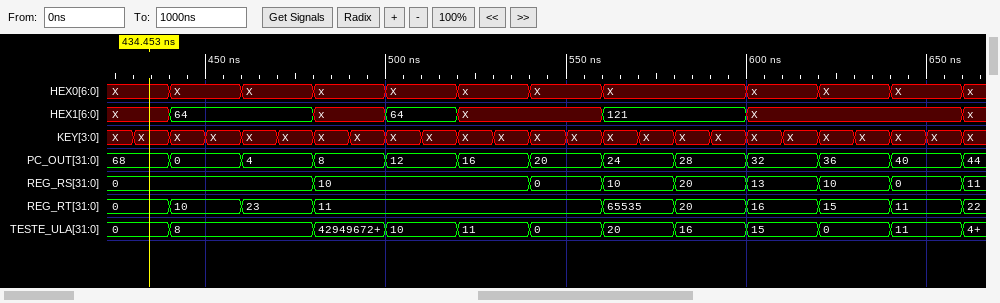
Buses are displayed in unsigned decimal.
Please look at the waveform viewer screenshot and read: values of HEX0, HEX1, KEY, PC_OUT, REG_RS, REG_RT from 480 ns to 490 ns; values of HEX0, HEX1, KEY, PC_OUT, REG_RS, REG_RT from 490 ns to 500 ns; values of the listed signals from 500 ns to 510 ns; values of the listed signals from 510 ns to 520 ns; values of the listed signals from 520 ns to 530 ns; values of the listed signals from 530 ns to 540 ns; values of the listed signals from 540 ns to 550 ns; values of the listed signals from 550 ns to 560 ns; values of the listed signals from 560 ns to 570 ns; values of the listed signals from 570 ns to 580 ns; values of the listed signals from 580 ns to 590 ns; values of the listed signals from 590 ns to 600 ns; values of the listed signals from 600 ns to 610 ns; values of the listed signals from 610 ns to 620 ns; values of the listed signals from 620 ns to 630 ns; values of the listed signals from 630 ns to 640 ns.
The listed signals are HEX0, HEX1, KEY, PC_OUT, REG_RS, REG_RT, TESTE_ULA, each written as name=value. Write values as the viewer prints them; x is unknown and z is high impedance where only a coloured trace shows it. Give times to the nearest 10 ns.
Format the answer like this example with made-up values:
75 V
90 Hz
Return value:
HEX0=x, HEX1=x, KEY=X, PC_OUT=8, REG_RS=10, REG_RT=11
HEX0=x, HEX1=x, KEY=X, PC_OUT=8, REG_RS=10, REG_RT=11
HEX0=X, HEX1=64, KEY=X, PC_OUT=12, REG_RS=10, REG_RT=11, TESTE_ULA=10
HEX0=X, HEX1=64, KEY=X, PC_OUT=12, REG_RS=10, REG_RT=11, TESTE_ULA=10
HEX0=x, HEX1=X, KEY=X, PC_OUT=16, REG_RS=10, REG_RT=11, TESTE_ULA=11
HEX0=x, HEX1=X, KEY=X, PC_OUT=16, REG_RS=10, REG_RT=11, TESTE_ULA=11
HEX0=X, HEX1=X, KEY=X, PC_OUT=20, REG_RS=0, REG_RT=11, TESTE_ULA=0
HEX0=X, HEX1=X, KEY=X, PC_OUT=20, REG_RS=0, REG_RT=11, TESTE_ULA=0
HEX0=X, HEX1=121, KEY=X, PC_OUT=24, REG_RS=10, REG_RT=65535, TESTE_ULA=20
HEX0=X, HEX1=121, KEY=X, PC_OUT=24, REG_RS=10, REG_RT=65535, TESTE_ULA=20
HEX0=X, HEX1=121, KEY=X, PC_OUT=28, REG_RS=20, REG_RT=20, TESTE_ULA=16
HEX0=X, HEX1=121, KEY=X, PC_OUT=28, REG_RS=20, REG_RT=20, TESTE_ULA=16
HEX0=x, HEX1=X, KEY=X, PC_OUT=32, REG_RS=13, REG_RT=16, TESTE_ULA=15
HEX0=x, HEX1=X, KEY=X, PC_OUT=32, REG_RS=13, REG_RT=16, TESTE_ULA=15
HEX0=X, HEX1=X, KEY=X, PC_OUT=36, REG_RS=10, REG_RT=15, TESTE_ULA=0
HEX0=X, HEX1=X, KEY=X, PC_OUT=36, REG_RS=10, REG_RT=15, TESTE_ULA=0
